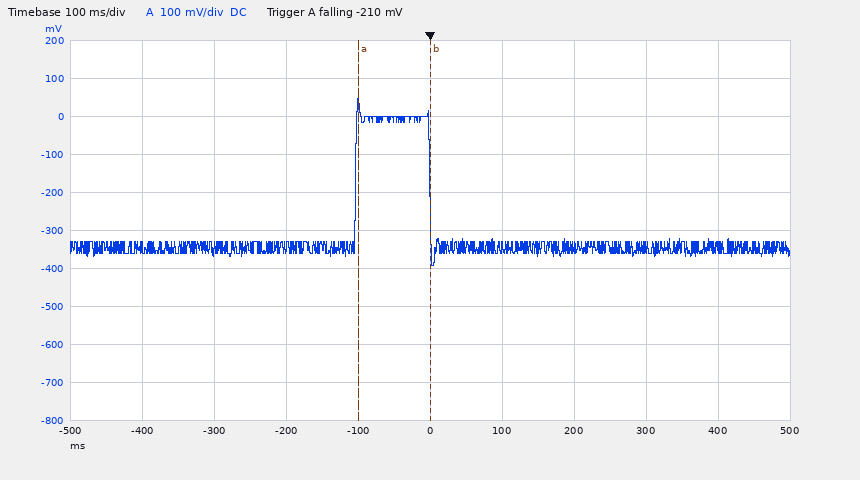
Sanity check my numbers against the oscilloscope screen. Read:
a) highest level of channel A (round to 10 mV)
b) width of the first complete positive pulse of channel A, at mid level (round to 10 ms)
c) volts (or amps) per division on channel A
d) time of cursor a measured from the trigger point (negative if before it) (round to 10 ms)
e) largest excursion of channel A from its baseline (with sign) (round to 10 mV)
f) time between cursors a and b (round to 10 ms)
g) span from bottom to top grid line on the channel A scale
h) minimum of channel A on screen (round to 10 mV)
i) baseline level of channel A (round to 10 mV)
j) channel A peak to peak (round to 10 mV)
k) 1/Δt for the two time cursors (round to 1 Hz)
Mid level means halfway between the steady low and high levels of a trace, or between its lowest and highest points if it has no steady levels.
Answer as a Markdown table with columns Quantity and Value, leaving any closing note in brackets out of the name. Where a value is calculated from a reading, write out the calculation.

| Quantity | Value |
|---|---|
| highest level of channel A | 50 mV |
| width of the first complete positive pulse of channel A, at mid level | 100 ms |
| volts (or amps) per division on channel A | 100 mV |
| time of cursor a measured from the trigger point (negative if before it) | -100 ms |
| largest excursion of channel A from its baseline (with sign) | 50 mV − (-340 mV) = +390 mV |
| time between cursors a and b | 100 ms |
| span from bottom to top grid line on the channel A scale | 1 V |
| minimum of channel A on screen | -390 mV |
| baseline level of channel A | -340 mV |
| channel A peak to peak | 50 mV − (-390 mV) = 440 mV |
| 1/Δt for the two time cursors | 1 / 100 ms ≈ 10 Hz |
